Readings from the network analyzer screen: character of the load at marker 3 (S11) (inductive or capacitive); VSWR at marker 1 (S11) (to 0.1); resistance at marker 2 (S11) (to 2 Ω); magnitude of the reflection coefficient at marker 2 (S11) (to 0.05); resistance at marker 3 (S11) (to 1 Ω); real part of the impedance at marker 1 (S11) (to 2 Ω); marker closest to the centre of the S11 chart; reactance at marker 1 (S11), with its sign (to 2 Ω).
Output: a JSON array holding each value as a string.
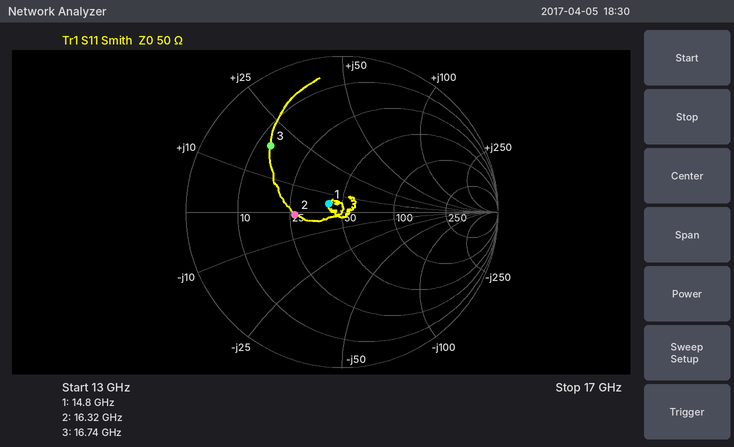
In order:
["inductive", "1.2", "26 Ω", "0.30", "13 Ω", "42 Ω", "marker 1", "+4 Ω"]
